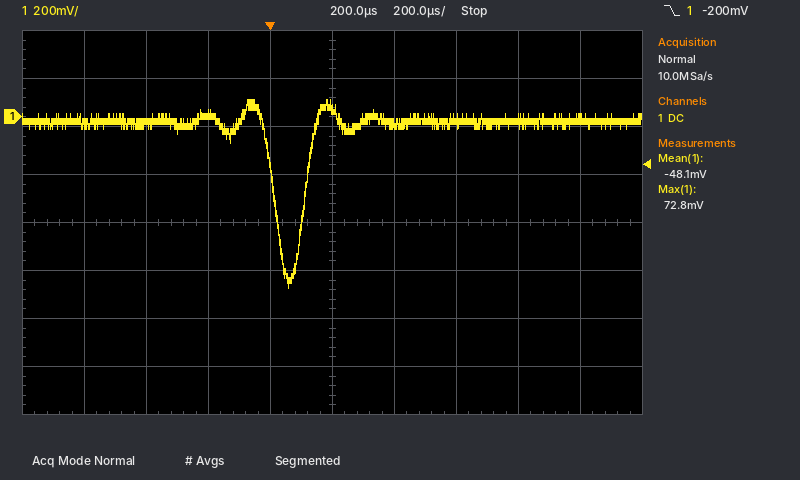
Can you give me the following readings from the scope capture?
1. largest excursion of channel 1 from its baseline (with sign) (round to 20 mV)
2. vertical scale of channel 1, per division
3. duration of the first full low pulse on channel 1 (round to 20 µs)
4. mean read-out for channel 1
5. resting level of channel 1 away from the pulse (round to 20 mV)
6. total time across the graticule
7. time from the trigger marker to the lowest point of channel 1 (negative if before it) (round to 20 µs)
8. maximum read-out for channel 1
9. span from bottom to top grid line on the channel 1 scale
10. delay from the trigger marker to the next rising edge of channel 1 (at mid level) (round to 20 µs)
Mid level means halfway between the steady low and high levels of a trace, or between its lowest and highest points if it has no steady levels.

-700 mV
200 mV
100 µs
-48.1 mV
-20 mV
2 ms
+60 µs
72.8 mV
1.6 V
120 µs
